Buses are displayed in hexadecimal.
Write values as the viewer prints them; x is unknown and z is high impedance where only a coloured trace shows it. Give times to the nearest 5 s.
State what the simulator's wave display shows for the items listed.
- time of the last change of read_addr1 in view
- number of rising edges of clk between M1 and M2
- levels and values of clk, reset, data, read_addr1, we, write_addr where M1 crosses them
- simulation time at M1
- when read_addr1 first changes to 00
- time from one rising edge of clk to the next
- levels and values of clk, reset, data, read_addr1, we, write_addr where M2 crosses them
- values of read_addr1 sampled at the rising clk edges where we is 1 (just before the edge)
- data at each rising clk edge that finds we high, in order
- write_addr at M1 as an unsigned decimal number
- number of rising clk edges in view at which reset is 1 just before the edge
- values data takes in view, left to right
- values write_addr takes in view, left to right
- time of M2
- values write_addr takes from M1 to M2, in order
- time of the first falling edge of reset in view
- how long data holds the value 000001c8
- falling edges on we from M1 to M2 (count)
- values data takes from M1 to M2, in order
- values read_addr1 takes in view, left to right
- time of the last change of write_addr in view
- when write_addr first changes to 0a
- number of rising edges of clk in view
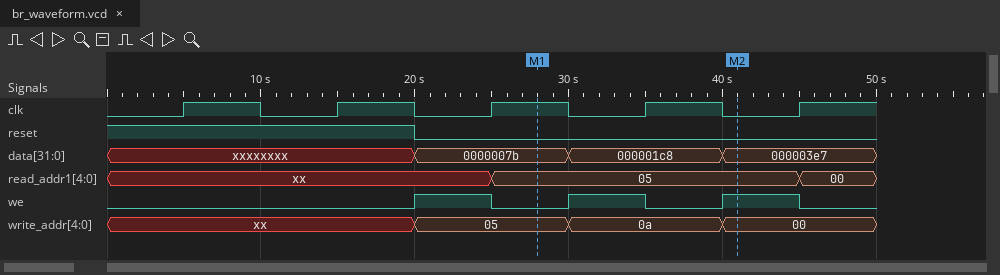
45 s
1
clk=1, reset=0, data=0000007b, read_addr1=05, we=0, write_addr=05
30 s
45 s
10 s
clk=0, reset=0, data=000003e7, read_addr1=05, we=1, write_addr=00
xx, 05, 05
0000007b, 000001c8, 000003e7
5
2
xxxxxxxx, 0000007b, 000001c8, 000003e7
xx, 05, 0a, 00
40 s
05, 0a, 00
20 s
10 s
1
0000007b, 000001c8, 000003e7
xx, 05, 00
40 s
30 s
5
